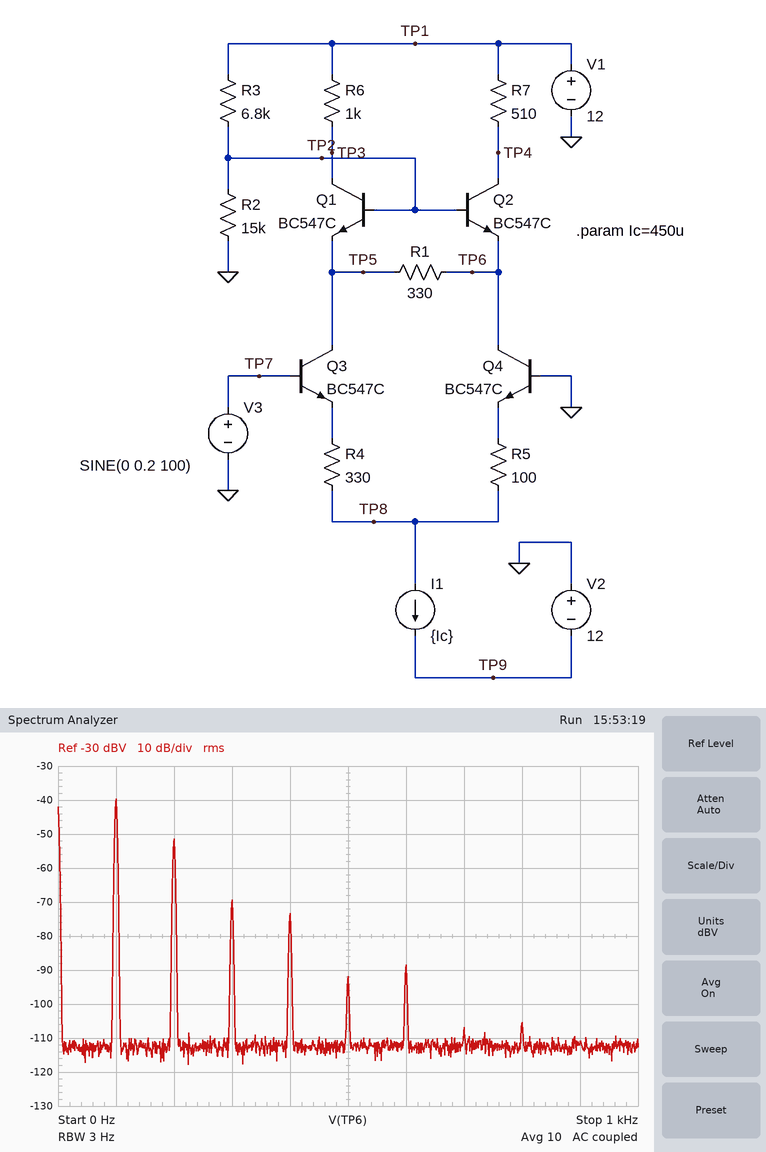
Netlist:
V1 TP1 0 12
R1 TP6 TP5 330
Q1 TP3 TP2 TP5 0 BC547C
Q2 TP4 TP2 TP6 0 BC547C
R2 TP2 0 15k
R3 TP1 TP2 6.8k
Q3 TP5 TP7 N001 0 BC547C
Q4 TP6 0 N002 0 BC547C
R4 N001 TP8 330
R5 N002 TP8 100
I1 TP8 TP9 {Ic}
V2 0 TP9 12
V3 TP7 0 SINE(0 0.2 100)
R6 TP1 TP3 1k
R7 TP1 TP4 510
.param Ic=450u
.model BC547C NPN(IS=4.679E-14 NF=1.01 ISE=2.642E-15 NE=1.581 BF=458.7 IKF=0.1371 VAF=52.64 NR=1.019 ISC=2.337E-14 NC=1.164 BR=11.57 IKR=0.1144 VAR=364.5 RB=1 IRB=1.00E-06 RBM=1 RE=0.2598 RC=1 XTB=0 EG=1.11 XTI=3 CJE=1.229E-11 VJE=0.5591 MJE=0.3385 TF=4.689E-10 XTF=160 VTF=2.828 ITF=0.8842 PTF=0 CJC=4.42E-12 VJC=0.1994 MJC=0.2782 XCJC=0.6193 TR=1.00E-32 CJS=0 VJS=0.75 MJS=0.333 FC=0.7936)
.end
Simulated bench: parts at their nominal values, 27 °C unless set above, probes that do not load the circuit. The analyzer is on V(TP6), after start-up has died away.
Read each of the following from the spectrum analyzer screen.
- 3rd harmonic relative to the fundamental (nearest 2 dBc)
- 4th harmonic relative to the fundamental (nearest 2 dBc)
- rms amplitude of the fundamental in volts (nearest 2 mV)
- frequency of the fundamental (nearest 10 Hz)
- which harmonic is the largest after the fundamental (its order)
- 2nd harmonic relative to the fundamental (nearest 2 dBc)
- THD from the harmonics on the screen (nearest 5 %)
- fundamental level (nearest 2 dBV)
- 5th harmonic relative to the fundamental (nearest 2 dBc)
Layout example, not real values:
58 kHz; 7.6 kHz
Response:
-30 dBc; -34 dBc; 10 mV; 100 Hz; 2; -12 dBc; 25 %; -40 dBV; -52 dBc
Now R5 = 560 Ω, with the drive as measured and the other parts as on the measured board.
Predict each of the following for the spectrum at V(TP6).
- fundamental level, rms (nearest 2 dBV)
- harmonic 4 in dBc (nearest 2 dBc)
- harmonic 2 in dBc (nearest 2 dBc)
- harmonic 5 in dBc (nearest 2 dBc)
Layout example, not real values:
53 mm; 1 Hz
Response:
-40 dBV; -42 dBc; -22 dBc; -50 dBc
